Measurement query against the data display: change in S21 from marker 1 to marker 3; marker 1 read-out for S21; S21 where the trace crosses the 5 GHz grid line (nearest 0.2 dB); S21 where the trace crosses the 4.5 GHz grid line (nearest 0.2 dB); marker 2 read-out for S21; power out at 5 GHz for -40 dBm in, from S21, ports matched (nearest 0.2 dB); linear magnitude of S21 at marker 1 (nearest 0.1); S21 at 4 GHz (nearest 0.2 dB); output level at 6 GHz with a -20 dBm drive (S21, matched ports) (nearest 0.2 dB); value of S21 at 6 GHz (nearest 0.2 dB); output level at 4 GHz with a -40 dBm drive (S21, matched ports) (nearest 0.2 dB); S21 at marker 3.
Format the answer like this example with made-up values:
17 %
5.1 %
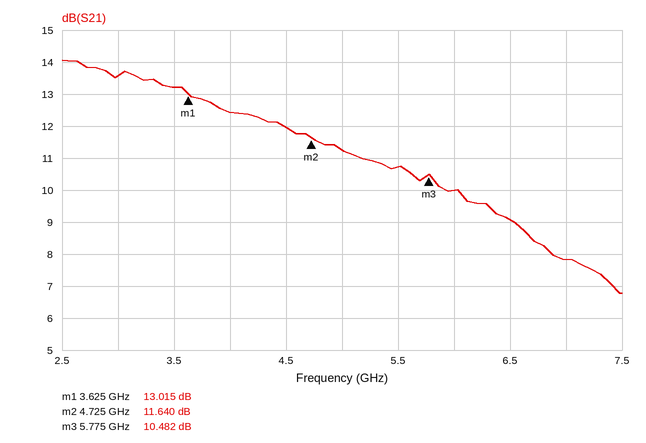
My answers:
-2.533 dB
13.015 dB
11.2 dB
12.0 dB
11.640 dB
-28.8 dBm
4.5
12.4 dB
-10.0 dBm
10.0 dB
-27.6 dBm
10.482 dB
